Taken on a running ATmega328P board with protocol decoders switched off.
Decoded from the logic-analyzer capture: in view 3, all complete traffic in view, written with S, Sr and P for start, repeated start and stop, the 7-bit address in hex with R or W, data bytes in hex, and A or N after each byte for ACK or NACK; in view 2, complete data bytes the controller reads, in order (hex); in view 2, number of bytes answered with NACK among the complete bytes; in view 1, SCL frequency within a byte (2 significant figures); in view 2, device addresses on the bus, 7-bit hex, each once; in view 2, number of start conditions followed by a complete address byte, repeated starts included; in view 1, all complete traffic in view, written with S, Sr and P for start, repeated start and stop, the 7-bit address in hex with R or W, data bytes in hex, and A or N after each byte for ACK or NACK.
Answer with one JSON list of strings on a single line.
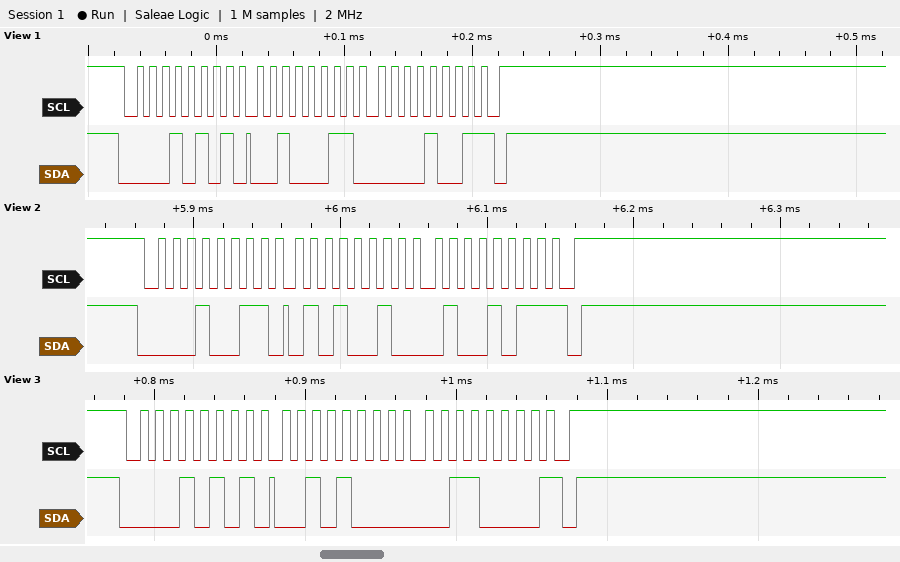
["S 0AR A 28 A 30 N P", "52 4B", "1", "100 kHz", "0x09", "1", "S 0AR A 23 A 09 N P"]
